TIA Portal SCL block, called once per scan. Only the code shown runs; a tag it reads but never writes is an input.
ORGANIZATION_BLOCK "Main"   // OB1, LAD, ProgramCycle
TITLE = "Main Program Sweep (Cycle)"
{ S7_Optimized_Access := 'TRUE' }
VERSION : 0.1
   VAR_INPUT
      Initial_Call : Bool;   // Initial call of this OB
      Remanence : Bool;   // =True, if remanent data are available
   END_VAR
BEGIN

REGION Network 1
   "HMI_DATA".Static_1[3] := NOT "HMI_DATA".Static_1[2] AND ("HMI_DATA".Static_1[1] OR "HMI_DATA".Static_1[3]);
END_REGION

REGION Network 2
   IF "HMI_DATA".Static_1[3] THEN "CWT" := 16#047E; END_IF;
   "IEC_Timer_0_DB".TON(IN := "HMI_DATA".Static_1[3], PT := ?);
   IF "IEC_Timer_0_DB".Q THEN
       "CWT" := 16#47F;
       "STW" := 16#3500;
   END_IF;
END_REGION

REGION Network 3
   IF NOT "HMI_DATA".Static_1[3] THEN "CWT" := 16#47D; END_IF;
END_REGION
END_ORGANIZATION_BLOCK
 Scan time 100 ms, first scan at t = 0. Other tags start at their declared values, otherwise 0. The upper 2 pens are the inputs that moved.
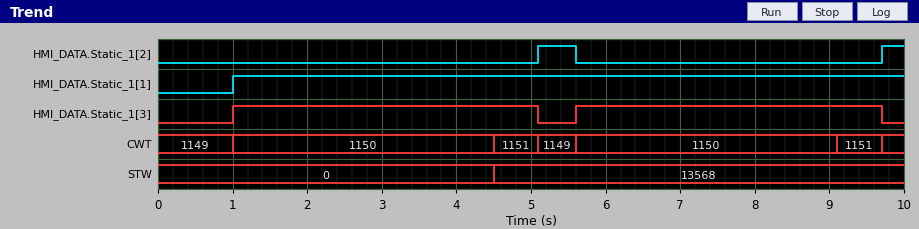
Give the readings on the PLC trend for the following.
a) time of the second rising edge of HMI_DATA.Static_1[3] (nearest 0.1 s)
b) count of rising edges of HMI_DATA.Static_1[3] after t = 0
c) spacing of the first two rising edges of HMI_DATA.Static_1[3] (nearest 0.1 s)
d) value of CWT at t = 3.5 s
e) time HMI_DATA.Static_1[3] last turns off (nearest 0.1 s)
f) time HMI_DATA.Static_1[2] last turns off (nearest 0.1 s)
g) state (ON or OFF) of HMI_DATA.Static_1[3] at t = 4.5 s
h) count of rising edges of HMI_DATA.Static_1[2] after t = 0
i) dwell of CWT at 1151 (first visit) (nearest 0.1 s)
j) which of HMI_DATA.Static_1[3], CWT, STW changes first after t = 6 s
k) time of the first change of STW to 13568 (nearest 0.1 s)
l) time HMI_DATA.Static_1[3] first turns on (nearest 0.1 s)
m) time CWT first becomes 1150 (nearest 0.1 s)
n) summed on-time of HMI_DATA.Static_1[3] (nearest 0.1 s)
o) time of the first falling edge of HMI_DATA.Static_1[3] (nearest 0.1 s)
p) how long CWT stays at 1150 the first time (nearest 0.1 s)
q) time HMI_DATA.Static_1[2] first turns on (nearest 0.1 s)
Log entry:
5.6 s
2
4.6 s
1150
9.7 s
5.6 s
ON
2
0.6 s
CWT
4.5 s
1.0 s
1.0 s
8.2 s
5.1 s
3.5 s
5.1 s
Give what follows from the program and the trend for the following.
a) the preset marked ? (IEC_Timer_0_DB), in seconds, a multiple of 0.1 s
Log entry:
3.5 s
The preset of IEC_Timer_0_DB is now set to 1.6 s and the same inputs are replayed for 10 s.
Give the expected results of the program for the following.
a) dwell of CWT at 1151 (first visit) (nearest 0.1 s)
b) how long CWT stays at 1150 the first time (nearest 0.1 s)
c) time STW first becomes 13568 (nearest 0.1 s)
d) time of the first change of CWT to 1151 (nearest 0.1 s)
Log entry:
2.5 s
1.6 s
2.6 s
2.6 s
